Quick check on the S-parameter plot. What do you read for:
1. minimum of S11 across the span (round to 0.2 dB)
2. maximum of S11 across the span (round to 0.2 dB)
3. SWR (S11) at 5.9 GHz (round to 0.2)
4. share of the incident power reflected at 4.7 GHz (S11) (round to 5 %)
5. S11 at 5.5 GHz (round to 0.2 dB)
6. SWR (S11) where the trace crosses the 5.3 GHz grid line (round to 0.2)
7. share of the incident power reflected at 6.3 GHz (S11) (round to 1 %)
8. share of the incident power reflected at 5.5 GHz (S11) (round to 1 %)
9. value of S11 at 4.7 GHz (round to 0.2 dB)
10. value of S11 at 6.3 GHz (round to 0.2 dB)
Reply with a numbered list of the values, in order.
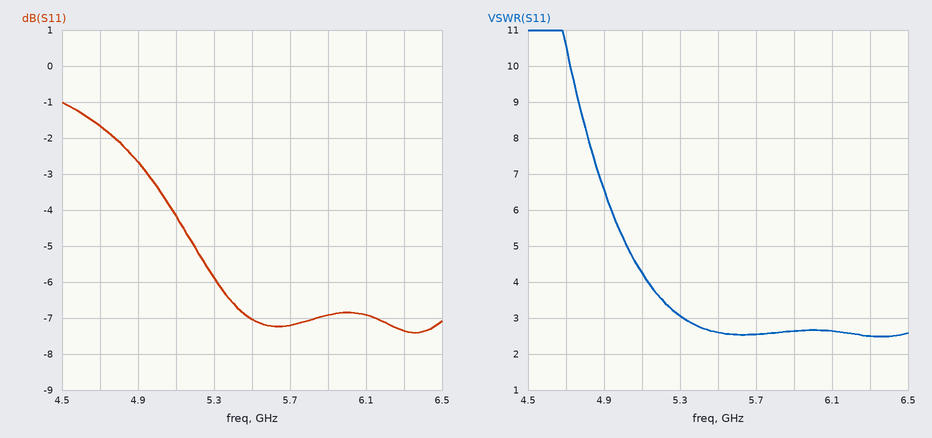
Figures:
1. -7.4 dB
2. -1.0 dB
3. 2.6
4. 70 %
5. -7.0 dB
6. 3.0
7. 18 %
8. 20 %
9. -1.6 dB
10. -7.4 dB
